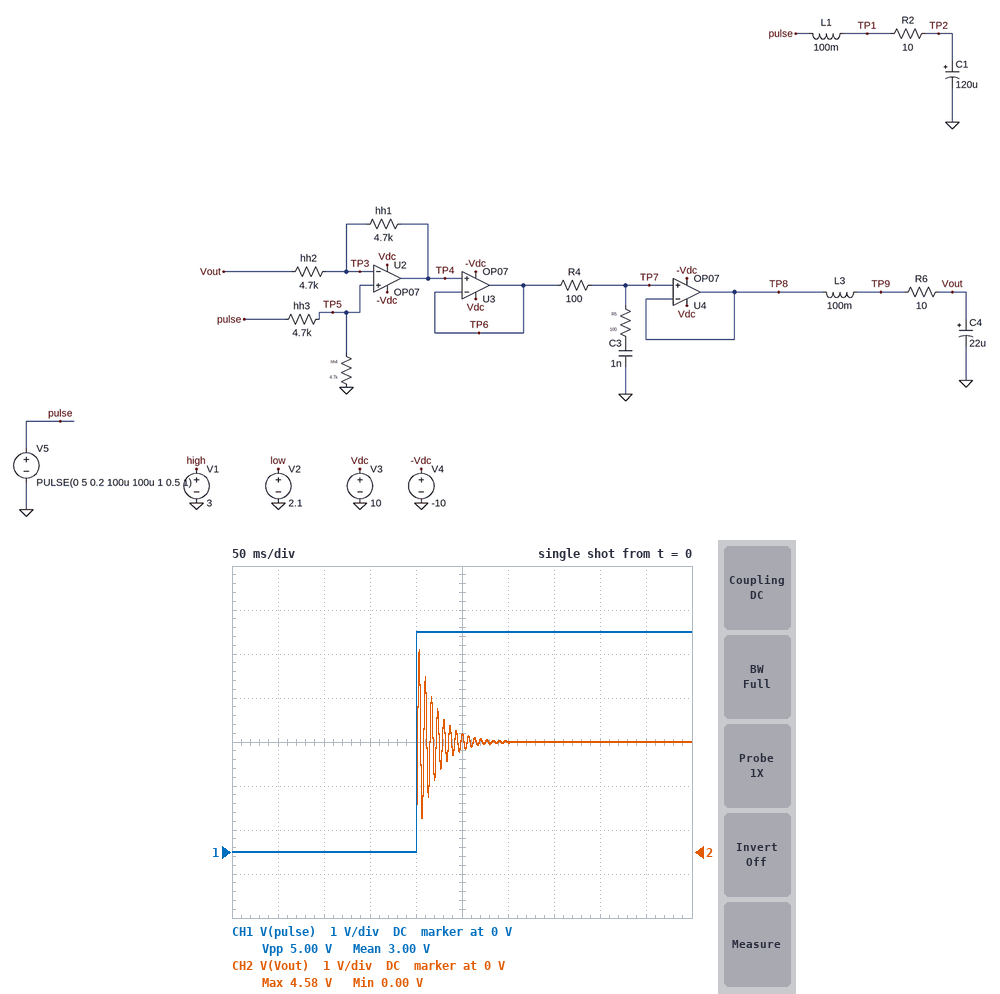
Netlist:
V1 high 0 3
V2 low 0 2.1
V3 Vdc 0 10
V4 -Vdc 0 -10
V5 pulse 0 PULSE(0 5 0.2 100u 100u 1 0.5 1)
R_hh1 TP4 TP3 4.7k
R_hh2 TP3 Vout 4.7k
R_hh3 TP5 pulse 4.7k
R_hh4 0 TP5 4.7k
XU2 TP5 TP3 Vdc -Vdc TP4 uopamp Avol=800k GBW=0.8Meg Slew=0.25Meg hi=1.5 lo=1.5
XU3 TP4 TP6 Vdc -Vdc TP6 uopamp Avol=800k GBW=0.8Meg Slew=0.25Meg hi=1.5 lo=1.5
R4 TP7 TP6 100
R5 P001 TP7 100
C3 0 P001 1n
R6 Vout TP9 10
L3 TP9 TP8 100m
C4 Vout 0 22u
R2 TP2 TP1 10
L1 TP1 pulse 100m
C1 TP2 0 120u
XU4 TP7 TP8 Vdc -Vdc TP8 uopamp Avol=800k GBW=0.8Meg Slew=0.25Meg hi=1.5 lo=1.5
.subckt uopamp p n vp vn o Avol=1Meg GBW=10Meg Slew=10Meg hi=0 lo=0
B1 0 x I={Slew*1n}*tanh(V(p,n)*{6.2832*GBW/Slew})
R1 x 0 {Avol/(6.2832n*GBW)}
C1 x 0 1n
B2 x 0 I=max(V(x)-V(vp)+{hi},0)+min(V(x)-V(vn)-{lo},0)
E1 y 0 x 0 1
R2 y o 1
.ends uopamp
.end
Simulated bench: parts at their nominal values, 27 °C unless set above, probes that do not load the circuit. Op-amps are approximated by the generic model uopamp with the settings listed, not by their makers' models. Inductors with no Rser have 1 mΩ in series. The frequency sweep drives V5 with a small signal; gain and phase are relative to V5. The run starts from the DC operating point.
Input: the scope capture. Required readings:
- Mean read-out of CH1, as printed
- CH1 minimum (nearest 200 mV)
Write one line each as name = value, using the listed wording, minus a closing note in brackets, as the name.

Mean read-out of CH1, as printed = 3.00 V
CH1 minimum = 0 V
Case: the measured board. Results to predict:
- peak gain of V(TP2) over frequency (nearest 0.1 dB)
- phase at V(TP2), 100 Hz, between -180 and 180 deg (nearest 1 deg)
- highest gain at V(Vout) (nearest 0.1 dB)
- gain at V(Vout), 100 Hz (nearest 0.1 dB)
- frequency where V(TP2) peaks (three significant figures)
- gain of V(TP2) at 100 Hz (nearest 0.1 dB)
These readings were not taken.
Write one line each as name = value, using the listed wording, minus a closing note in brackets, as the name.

peak gain of V(TP2) over frequency = 9.3 dB
phase at V(TP2), 100 Hz, between -180 and 180 deg = -169 deg
highest gain at V(Vout) = 12.8 dB
gain at V(Vout), 100 Hz = -1.2 dB
frequency where V(TP2) peaks = 44.5 Hz
gain of V(TP2) at 100 Hz = -11.6 dB
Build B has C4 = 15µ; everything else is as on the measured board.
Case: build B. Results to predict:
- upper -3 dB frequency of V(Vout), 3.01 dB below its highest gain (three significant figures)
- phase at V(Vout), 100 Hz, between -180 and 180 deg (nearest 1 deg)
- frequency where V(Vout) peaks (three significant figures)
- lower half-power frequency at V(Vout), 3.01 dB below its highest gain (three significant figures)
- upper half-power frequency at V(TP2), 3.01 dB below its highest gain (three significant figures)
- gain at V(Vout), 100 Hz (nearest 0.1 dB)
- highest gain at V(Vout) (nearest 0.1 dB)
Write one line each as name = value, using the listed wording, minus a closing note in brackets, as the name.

upper -3 dB frequency of V(Vout), 3.01 dB below its highest gain = 192 Hz
phase at V(Vout), 100 Hz, between -180 and 180 deg = -4 deg
frequency where V(Vout) peaks = 183 Hz
lower half-power frequency at V(Vout), 3.01 dB below its highest gain = 174 Hz
upper half-power frequency at V(TP2), 3.01 dB below its highest gain = 52.0 Hz
gain at V(Vout), 100 Hz = -3.0 dB
highest gain at V(Vout) = 14.1 dB
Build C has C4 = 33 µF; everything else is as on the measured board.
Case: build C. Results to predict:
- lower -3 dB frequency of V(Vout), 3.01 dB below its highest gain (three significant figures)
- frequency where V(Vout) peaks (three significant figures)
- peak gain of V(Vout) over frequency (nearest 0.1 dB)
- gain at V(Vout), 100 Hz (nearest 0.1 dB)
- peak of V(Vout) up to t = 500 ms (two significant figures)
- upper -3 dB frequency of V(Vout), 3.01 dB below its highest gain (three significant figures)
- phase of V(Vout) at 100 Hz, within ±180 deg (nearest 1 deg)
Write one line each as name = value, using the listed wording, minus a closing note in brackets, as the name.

lower -3 dB frequency of V(Vout), 3.01 dB below its highest gain = 115 Hz
frequency where V(Vout) peaks = 123 Hz
peak gain of V(Vout) over frequency = 11.3 dB
gain at V(Vout), 100 Hz = 2.7 dB
peak of V(Vout) up to t = 500 ms = 4.5 V
upper -3 dB frequency of V(Vout), 3.01 dB below its highest gain = 132 Hz
phase of V(Vout) at 100 Hz, within ±180 deg = -17 deg
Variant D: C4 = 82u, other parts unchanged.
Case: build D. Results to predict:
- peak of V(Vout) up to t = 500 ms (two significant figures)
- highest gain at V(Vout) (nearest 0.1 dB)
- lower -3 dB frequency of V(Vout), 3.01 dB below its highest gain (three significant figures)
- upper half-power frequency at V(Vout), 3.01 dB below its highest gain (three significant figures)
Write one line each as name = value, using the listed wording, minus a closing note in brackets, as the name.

peak of V(Vout) up to t = 500 ms = 4.3 V
highest gain at V(Vout) = 7.7 dB
lower -3 dB frequency of V(Vout), 3.01 dB below its highest gain = 69.1 Hz
upper half-power frequency at V(Vout), 3.01 dB below its highest gain = 85.6 Hz
